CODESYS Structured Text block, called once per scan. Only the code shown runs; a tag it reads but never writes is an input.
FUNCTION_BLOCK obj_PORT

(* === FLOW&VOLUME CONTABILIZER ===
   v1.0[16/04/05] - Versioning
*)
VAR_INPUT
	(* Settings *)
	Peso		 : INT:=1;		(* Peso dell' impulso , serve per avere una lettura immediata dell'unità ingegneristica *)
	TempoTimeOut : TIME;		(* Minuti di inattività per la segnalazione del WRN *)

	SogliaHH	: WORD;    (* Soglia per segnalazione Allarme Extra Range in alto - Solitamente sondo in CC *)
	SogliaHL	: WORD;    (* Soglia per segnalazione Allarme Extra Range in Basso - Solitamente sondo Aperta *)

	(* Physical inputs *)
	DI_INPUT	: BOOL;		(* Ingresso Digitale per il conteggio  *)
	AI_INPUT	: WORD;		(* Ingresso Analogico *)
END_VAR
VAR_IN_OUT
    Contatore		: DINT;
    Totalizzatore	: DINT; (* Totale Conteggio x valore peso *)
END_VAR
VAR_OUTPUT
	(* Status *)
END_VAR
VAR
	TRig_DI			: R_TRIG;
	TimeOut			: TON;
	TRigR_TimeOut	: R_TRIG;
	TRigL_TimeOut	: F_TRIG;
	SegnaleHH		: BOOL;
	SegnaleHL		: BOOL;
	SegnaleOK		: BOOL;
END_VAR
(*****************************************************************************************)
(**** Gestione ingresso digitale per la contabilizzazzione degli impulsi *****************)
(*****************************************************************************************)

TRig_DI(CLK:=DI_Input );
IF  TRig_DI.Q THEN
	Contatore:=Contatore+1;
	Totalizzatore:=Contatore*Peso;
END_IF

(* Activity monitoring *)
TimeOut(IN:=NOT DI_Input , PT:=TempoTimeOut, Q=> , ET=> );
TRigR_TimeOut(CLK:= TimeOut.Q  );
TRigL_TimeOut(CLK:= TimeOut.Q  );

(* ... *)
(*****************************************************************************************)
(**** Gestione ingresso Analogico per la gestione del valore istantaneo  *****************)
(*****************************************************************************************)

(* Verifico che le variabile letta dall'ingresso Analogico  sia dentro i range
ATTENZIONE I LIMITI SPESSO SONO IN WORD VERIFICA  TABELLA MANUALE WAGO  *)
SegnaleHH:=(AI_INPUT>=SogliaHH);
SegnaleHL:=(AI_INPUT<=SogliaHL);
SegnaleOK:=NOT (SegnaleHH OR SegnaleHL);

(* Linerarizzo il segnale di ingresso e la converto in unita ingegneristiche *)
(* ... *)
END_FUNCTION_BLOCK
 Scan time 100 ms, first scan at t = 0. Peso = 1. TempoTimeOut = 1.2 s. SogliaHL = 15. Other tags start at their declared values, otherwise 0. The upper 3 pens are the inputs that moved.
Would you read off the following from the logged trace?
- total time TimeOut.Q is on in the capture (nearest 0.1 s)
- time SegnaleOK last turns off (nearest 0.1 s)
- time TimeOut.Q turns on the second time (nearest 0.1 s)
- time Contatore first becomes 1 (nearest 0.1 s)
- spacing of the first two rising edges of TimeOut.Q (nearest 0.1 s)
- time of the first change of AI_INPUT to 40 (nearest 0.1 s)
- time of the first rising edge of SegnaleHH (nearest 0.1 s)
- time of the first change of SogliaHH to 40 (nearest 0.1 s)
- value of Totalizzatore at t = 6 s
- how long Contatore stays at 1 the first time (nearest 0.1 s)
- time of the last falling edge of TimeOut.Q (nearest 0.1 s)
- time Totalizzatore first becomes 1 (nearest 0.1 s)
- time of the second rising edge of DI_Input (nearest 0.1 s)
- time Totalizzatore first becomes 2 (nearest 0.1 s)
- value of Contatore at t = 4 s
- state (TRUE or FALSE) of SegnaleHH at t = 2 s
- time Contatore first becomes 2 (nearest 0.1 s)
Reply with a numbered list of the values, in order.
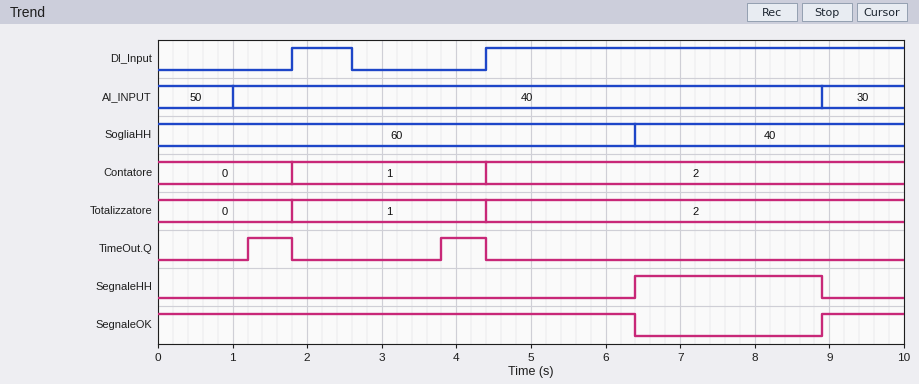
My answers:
1. 1.2 s
2. 6.4 s
3. 3.8 s
4. 1.8 s
5. 2.6 s
6. 1.0 s
7. 6.4 s
8. 6.4 s
9. 2
10. 2.6 s
11. 4.4 s
12. 1.8 s
13. 4.4 s
14. 4.4 s
15. 1
16. FALSE
17. 4.4 s
